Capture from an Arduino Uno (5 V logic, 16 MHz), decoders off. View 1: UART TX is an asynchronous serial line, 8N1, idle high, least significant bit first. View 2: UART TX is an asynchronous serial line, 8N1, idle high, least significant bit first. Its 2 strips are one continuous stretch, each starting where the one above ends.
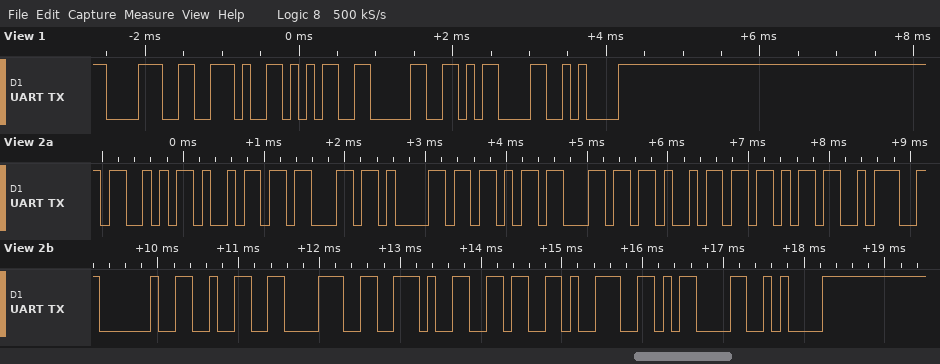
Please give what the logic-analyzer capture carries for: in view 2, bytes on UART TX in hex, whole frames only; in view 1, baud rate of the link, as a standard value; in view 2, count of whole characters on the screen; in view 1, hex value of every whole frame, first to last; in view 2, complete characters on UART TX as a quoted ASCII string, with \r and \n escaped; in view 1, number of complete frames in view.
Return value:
0x53 0x69 0x63 0x61 0x6B 0x6C 0x69 0x6B 0x3A 0x20 0x32 0x38 0x2E 0x36 0x39 0x0D 0x0A
9600 baud
17
38 2E 35 30 0D 0A
"Sicaklik: 28.69\r\n"
6
